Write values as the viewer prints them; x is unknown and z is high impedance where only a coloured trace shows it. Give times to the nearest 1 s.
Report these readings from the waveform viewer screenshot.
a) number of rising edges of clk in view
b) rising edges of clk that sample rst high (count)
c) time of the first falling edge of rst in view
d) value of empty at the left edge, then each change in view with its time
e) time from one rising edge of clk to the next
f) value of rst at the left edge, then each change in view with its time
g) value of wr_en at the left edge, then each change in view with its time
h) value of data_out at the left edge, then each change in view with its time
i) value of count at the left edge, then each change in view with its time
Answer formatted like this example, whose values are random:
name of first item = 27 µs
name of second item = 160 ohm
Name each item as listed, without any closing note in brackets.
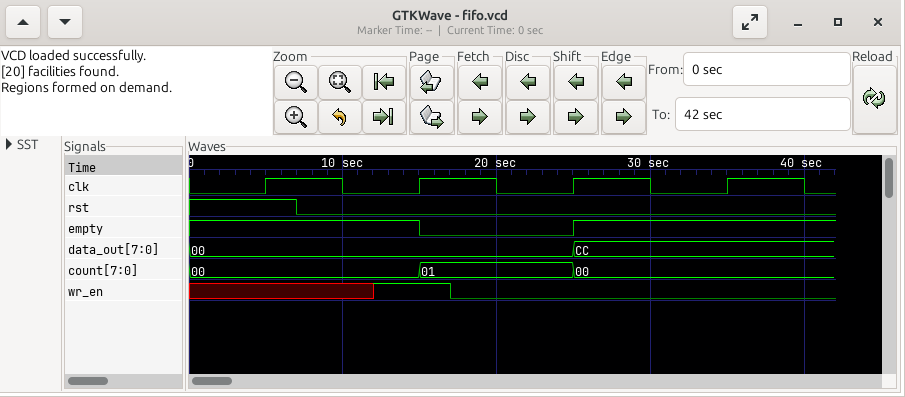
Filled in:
number of rising edges of clk in view = 4
rising edges of clk that sample rst high = 1
time of the first falling edge of rst in view = 7 s
value of empty at the left edge, then each change in view with its time = 1, 0 at 15 s, 1 at 25 s
time from one rising edge of clk to the next = 10 s
value of rst at the left edge, then each change in view with its time = 1, 0 at 7 s
value of wr_en at the left edge, then each change in view with its time = x, 1 at 12 s, 0 at 17 s
value of data_out at the left edge, then each change in view with its time = 00, CC at 25 s
value of count at the left edge, then each change in view with its time = 00, 01 at 15 s, 00 at 25 s
